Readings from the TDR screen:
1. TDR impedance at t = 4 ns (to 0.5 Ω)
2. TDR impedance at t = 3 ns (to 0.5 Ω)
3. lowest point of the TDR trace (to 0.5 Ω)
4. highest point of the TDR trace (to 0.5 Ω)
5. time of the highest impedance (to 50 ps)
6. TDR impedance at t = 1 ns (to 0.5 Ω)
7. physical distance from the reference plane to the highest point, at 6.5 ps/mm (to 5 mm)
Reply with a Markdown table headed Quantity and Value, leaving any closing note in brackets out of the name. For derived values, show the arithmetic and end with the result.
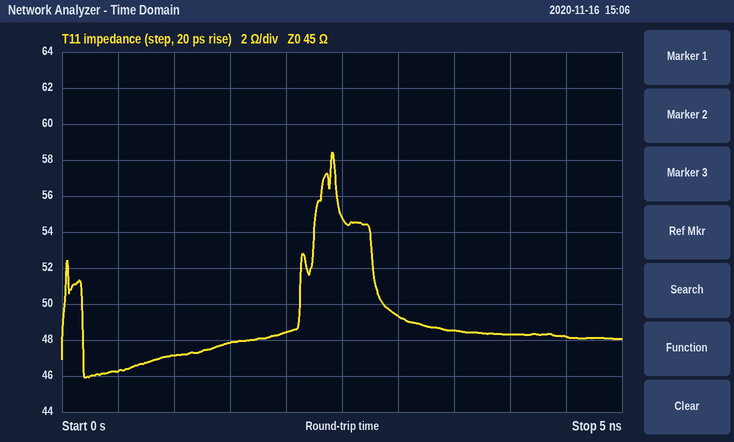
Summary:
| Quantity | Value |
|---|---|
| TDR impedance at t = 4 ns | 48.5 Ω |
| TDR impedance at t = 3 ns | 49.5 Ω |
| lowest point of the TDR trace | 46.0 Ω |
| highest point of the TDR trace | 58.5 Ω |
| time of the highest impedance | 2.40 ns |
| TDR impedance at t = 1 ns | 47.0 Ω |
| physical distance from the reference plane to the highest point, at 6.5 ps/mm | 2.40 ns / 2 / 6.5 ps/mm ≈ 185 mm |
